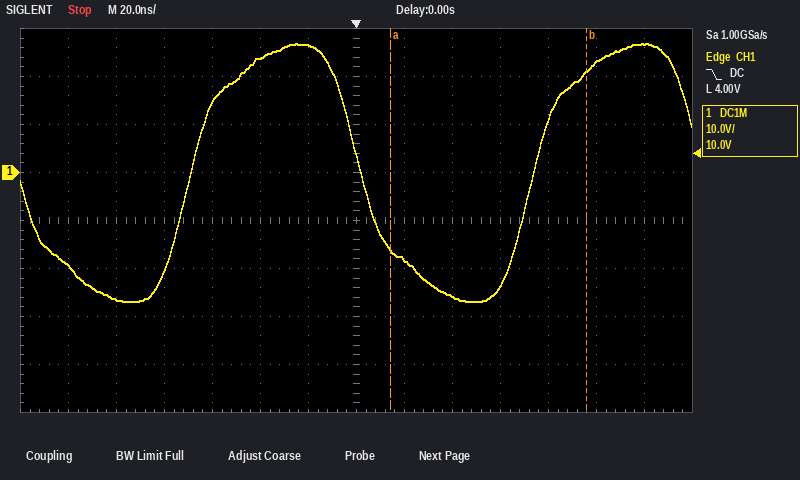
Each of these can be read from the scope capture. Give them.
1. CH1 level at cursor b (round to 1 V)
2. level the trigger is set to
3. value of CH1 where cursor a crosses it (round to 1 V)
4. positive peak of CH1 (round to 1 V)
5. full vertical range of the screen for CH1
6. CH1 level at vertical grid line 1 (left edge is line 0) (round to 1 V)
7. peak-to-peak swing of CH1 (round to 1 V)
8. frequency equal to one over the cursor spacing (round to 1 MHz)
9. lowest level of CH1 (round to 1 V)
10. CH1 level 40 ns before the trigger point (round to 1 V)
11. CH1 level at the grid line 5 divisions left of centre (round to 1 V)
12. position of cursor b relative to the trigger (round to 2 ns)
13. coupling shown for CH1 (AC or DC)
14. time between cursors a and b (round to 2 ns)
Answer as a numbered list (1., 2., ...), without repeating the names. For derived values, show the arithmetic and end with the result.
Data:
1. 21 V
2. 4.00 V
3. -16 V
4. 27 V
5. 80 V
6. -19 V
7. 27 V − (-27 V) = 54 V
8. 1 / 82 ns ≈ 12 MHz
9. -27 V
10. 24 V
11. -26 V
12. +96 ns
13. DC
14. 82 ns
